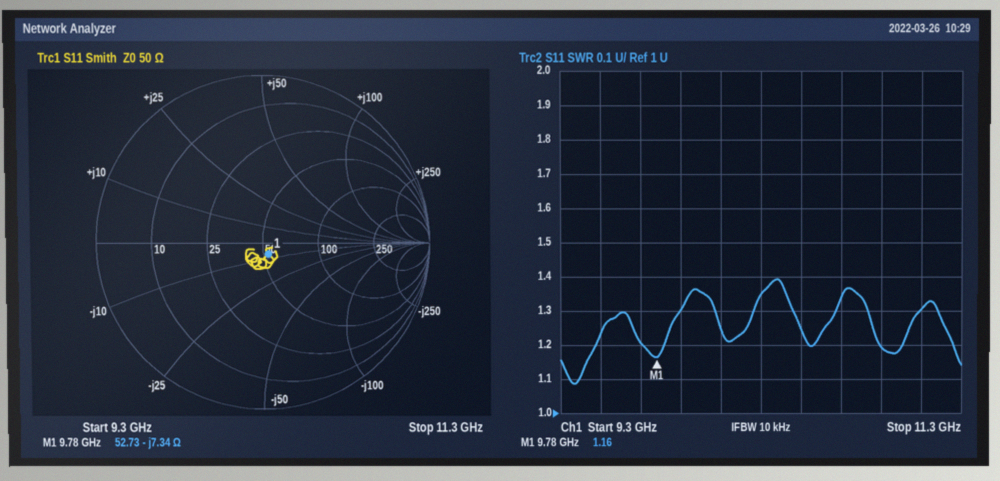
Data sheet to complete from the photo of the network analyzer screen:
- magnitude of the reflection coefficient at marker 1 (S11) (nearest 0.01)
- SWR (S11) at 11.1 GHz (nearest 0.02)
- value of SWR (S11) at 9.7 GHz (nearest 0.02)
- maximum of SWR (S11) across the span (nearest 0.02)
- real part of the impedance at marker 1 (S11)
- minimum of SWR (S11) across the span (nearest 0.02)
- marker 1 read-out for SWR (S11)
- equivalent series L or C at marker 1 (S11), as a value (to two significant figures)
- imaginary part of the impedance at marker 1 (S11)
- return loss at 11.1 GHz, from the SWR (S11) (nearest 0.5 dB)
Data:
0.08
1.30
1.20
1.40
52.73 Ω
1.08
1.16
2.2 pF
-7.34 Ω
17.5 dB
